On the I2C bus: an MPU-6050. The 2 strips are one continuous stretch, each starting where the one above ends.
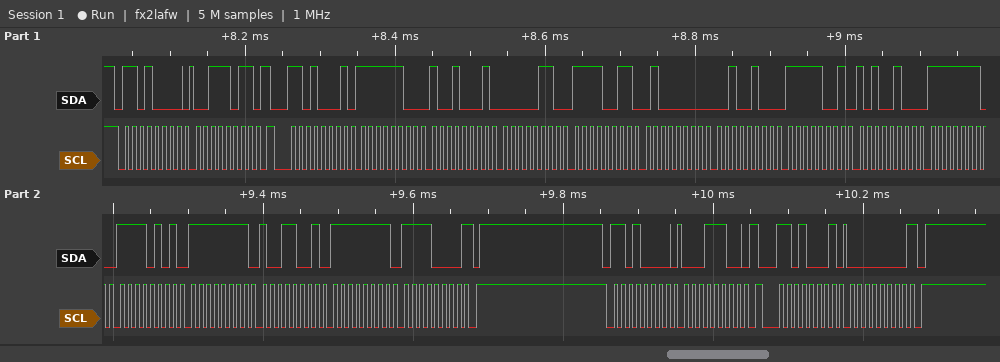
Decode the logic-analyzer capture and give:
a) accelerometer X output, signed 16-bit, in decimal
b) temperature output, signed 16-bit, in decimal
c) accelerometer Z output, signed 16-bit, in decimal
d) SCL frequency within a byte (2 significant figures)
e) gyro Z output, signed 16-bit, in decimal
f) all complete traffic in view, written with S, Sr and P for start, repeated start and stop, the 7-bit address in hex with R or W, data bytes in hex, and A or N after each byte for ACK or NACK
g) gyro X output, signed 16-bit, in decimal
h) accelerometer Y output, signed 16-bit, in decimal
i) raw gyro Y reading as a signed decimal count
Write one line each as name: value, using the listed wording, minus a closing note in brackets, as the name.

accelerometer X output, signed 16-bit, in decimal: -879
temperature output, signed 16-bit, in decimal: -1628
accelerometer Z output, signed 16-bit, in decimal: 16420
SCL frequency within a byte: 100 kHz
gyro Z output, signed 16-bit, in decimal: -16
all complete traffic in view, written with S, Sr and P for start, repeated start and stop, the 7-bit address in hex with R or W, data bytes in hex, and A or N after each byte for ACK or NACK: S 68W A 3B A Sr 68R A FC A 91 A 06 A F3 A 40 A 24 A F9 A A4 A FE A F5 A FF A 99 A FF A F0 N P S 68W A 1C A Sr 68R A 00 N P
gyro X output, signed 16-bit, in decimal: -267
accelerometer Y output, signed 16-bit, in decimal: 1779
raw gyro Y reading as a signed decimal count: -103
